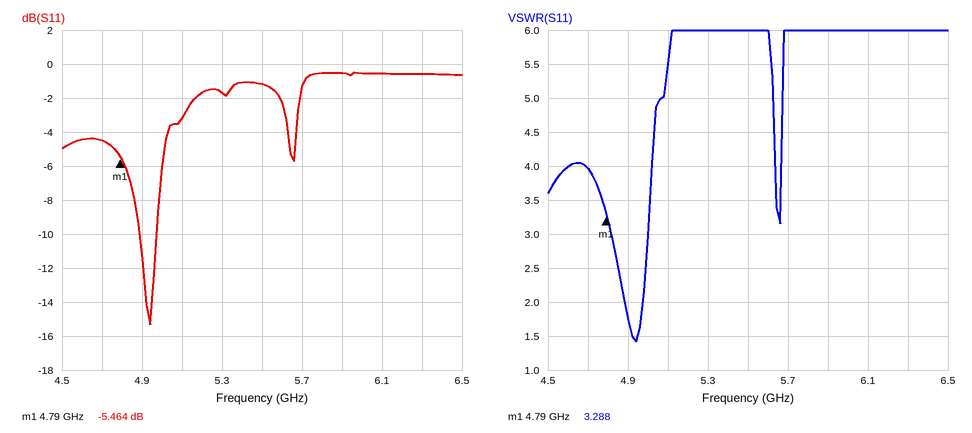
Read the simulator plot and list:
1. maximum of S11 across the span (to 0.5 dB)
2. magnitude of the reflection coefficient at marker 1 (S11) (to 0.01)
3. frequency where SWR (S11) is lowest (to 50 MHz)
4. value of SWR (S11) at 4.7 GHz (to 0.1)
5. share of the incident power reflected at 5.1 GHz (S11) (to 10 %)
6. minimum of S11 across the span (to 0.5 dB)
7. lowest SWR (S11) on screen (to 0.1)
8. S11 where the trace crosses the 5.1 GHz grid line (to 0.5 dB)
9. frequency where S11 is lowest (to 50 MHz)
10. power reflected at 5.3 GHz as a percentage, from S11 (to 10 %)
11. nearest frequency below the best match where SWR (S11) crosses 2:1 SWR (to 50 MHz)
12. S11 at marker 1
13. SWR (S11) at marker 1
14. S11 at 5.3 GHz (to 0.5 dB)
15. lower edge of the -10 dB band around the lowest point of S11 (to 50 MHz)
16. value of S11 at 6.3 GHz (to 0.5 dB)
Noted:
-0.5 dB
0.53
4.95 GHz
4.0
50 %
-15.5 dB
1.4
-3.0 dB
4.95 GHz
70 %
4.90 GHz
-5.464 dB
3.288
-1.5 dB
4.90 GHz
-0.5 dB
